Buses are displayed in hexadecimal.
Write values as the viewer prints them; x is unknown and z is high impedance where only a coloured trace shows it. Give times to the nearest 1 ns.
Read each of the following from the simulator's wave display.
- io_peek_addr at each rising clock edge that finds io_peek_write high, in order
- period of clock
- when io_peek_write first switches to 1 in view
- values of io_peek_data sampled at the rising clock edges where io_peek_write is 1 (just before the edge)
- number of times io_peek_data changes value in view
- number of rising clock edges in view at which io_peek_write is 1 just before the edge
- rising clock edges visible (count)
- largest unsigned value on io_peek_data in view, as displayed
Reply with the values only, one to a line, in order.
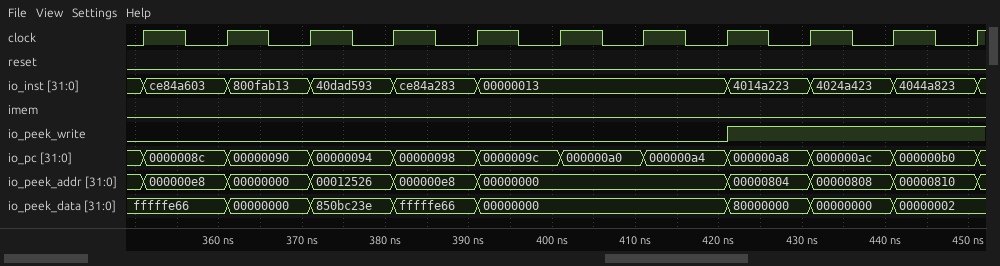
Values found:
00000804, 00000808, 00000810
10 ns
421 ns
80000000, 00000000, 00000002
7
3
11
fffffe66
